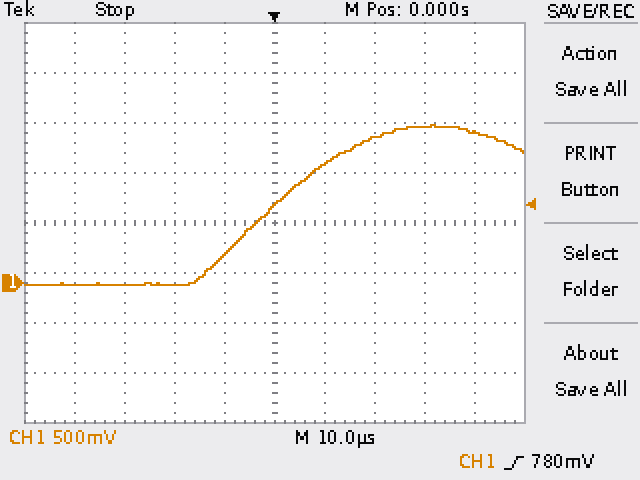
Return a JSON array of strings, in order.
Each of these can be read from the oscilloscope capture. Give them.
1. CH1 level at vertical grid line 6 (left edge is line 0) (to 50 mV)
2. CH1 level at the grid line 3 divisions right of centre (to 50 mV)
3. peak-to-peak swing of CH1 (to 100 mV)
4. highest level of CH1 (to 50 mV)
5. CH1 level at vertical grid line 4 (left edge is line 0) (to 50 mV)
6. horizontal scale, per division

["1.20 V", "1.55 V", "1.60 V", "1.60 V", "300 mV", "10 µs"]
